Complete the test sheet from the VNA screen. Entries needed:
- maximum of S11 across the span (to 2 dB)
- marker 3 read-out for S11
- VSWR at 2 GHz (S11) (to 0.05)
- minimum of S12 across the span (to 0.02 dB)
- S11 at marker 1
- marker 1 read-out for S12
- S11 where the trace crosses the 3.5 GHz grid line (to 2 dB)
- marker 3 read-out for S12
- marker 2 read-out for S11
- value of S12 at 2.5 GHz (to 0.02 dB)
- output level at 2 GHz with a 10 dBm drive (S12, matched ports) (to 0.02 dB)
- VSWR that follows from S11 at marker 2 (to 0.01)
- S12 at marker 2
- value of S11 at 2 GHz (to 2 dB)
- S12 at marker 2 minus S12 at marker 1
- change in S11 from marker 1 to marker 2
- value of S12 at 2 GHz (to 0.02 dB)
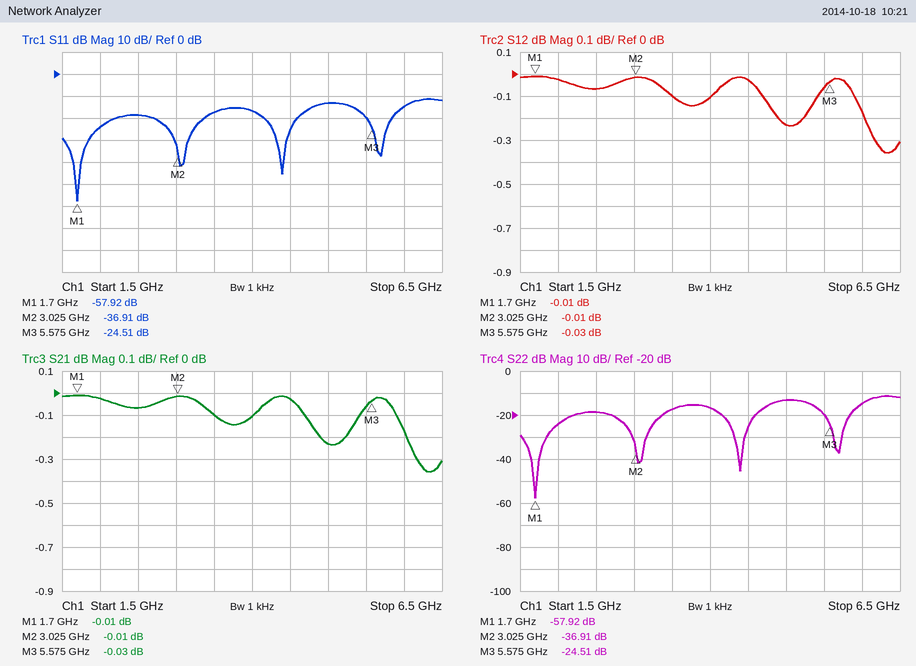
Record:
-12 dB
-24.51 dB
1.15
-0.36 dB
-57.92 dB
-0.01 dB
-18 dB
-0.03 dB
-36.91 dB
-0.06 dB
9.98 dBm
1.03
-0.01 dB
-24 dB
0.00 dB
21.01 dB
-0.02 dB
